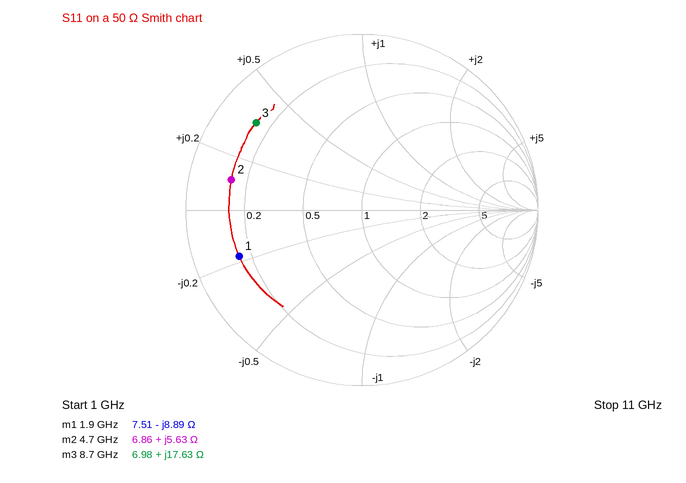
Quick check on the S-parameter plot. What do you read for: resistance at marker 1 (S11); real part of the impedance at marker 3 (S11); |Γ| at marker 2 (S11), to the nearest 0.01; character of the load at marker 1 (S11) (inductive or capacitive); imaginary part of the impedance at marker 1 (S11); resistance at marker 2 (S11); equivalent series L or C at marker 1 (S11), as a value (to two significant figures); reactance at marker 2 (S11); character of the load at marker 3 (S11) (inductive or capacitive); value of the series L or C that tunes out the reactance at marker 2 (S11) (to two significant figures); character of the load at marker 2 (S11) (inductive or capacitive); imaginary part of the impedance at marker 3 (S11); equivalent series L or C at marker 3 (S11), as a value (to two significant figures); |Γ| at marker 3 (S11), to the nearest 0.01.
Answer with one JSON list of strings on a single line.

["7.51 Ω", "6.98 Ω", "0.76", "capacitive", "-8.89 Ω", "6.86 Ω", "9.4 pF", "+5.63 Ω", "inductive", "6.0 pF", "inductive", "+17.63 Ω", "320 pH", "0.78"]
